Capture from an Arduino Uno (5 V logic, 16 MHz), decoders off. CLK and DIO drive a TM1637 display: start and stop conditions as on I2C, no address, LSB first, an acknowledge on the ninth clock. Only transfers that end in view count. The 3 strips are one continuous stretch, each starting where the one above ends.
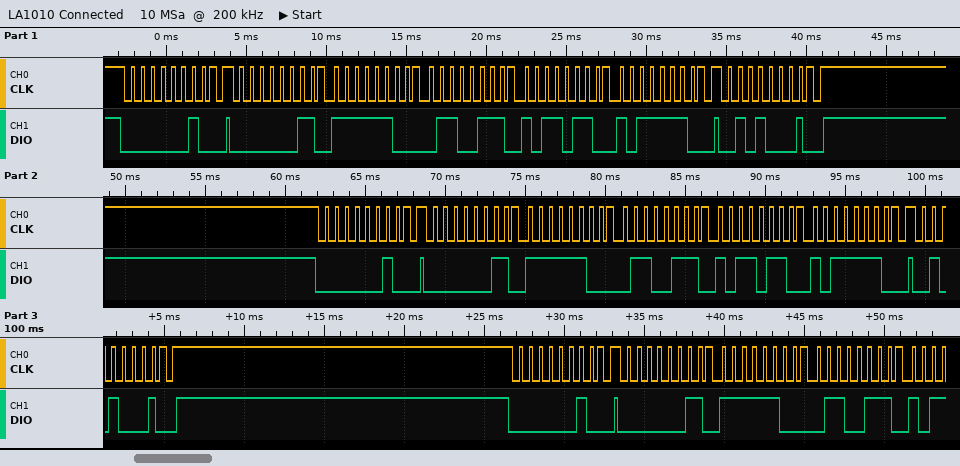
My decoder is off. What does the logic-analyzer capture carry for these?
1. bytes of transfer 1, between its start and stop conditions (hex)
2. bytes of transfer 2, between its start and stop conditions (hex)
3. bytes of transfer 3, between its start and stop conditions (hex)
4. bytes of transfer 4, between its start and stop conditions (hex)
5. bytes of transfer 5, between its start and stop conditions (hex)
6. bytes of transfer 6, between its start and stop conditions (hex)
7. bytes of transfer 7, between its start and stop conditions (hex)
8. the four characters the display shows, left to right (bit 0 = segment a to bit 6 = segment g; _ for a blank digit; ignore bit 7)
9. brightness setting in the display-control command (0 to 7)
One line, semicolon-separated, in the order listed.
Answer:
40; C0 3F E6 6D 7D; 8A; 40; C0 3F E6 6D 7D; 8A; 40; 0456; 2
